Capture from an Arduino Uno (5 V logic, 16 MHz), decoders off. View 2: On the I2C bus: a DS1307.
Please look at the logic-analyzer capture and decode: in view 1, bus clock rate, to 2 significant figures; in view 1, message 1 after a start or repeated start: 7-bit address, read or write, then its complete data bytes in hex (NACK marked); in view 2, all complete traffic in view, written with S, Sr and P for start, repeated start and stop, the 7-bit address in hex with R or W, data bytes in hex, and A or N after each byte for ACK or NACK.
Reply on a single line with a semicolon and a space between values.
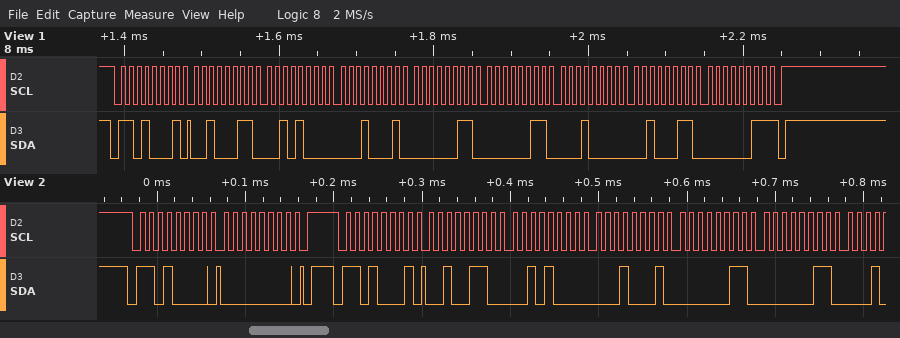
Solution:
100 kHz; 0x68 read: 23 28 11 03 03 10 23 03 NACK; S 68W A 00 A P S 68R A 26 A 28 A 11 A 03 A 03 A
